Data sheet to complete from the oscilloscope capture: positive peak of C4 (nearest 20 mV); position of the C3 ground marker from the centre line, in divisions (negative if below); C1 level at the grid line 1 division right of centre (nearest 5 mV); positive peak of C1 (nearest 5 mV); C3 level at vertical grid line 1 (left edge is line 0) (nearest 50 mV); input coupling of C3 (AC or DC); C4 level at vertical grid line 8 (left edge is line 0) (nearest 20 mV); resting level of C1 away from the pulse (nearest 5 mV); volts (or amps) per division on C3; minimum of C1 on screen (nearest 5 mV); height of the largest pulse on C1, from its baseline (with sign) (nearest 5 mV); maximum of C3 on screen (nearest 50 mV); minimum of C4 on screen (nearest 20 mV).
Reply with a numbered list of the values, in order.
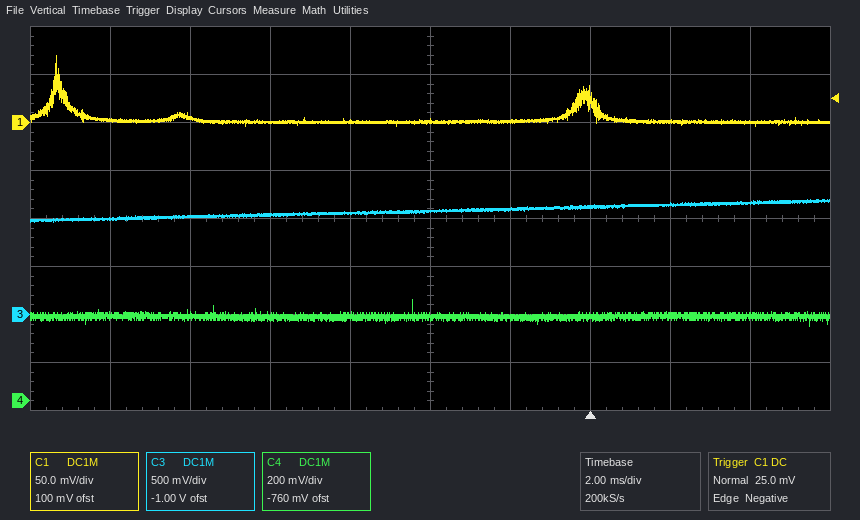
1. 420 mV
2. -2.0 div
3. 0 mV
4. 70 mV
5. 1.00 V
6. DC
7. 360 mV
8. 0 mV
9. 500 mV
10. -5 mV
11. +70 mV
12. 1.20 V
13. 320 mV
